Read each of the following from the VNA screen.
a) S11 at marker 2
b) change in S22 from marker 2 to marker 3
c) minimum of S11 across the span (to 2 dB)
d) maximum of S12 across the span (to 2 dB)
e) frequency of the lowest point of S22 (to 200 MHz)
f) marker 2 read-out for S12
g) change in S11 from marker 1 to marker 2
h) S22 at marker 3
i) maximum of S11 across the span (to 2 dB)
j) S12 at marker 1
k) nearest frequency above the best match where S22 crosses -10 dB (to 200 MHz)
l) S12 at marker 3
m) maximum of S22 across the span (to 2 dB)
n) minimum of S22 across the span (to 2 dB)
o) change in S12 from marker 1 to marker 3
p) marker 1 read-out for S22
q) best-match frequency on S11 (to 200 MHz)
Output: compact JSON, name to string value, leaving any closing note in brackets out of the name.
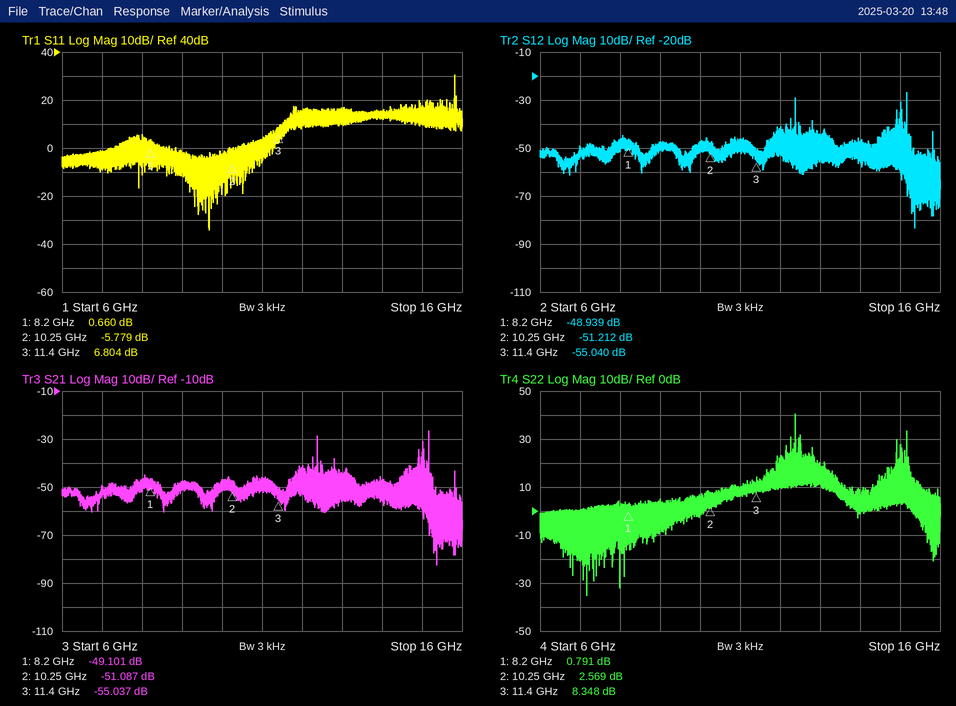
{"S11 at marker 2": "-5.779 dB", "change in S22 from marker 2 to marker 3": "5.779 dB", "minimum of S11 across the span": "-34 dB", "maximum of S12 across the span": "-26 dB", "frequency of the lowest point of S22": "7.2 GHz", "marker 2 read-out for S12": "-51.212 dB", "change in S11 from marker 1 to marker 2": "-6.439 dB", "S22 at marker 3": "8.348 dB", "maximum of S11 across the span": "30 dB", "S12 at marker 1": "-48.939 dB", "nearest frequency above the best match where S22 crosses -10 dB": "7.2 GHz", "S12 at marker 3": "-55.040 dB", "maximum of S22 across the span": "40 dB", "minimum of S22 across the span": "-36 dB", "change in S12 from marker 1 to marker 3": "-6.101 dB", "marker 1 read-out for S22": "0.791 dB", "best-match frequency on S11": "9.6 GHz"}
